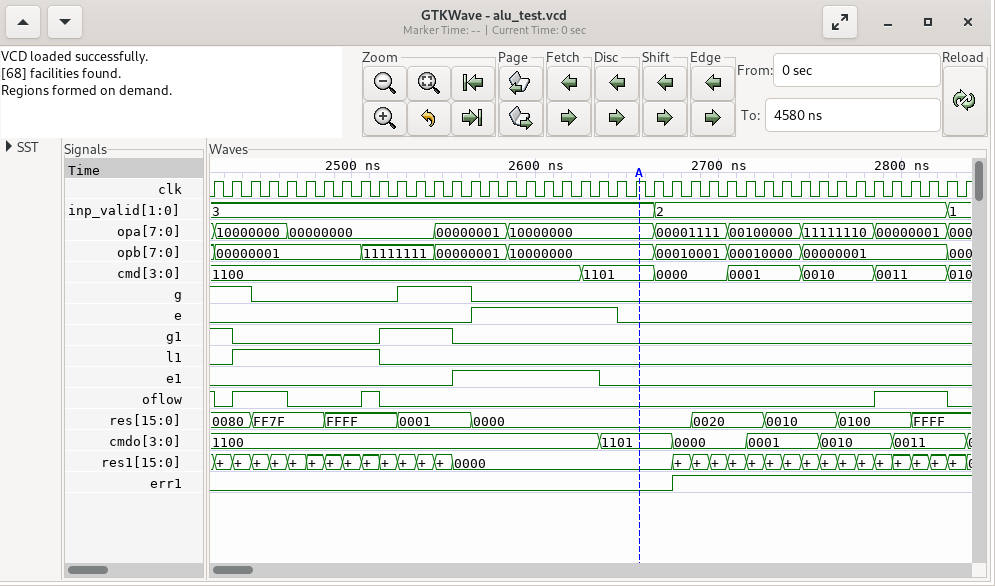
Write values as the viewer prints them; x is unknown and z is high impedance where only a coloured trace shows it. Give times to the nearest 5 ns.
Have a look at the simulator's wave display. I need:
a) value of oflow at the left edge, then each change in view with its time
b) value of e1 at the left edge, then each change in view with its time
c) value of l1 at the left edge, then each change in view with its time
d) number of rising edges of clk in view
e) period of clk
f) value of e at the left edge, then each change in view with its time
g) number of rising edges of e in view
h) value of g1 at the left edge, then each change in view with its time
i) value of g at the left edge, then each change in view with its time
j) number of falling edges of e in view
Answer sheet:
1, 0 at 2425 ns, 1 at 2435 ns, 0 at 2465 ns, 1 at 2505 ns, 0 at 2515 ns, 1 at 2785 ns, 0 at 2825 ns
0, 1 at 2555 ns, 0 at 2635 ns
0, 1 at 2435 ns, 0 at 2515 ns
42
10 ns
0, 1 at 2565 ns, 0 at 2645 ns
1
1, 0 at 2435 ns, 1 at 2515 ns, 0 at 2555 ns
1, 0 at 2445 ns, 1 at 2525 ns, 0 at 2565 ns
1
